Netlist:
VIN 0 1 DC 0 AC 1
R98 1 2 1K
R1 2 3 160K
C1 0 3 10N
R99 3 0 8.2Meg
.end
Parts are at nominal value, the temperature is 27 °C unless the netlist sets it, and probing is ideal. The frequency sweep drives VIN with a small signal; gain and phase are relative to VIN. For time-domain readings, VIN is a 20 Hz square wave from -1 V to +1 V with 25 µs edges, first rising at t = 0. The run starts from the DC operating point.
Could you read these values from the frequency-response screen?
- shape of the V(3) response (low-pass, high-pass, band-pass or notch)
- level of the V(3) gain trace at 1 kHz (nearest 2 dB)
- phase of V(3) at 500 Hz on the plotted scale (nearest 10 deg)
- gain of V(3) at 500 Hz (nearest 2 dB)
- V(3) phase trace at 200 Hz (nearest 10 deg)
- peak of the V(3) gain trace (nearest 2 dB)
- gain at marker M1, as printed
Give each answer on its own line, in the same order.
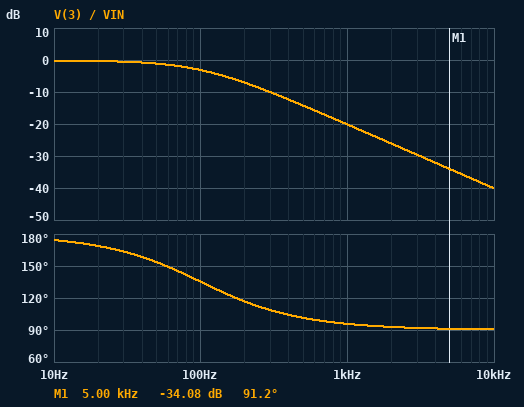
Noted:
low-pass
-20 dB
100 deg
-14 dB
120 deg
0 dB
-34.08 dB
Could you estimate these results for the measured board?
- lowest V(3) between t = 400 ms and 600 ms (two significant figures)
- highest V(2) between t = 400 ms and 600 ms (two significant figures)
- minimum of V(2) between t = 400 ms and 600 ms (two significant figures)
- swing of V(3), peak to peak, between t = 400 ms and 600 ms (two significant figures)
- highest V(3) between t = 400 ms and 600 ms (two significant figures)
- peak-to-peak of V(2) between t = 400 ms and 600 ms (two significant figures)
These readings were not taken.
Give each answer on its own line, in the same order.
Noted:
-980 mV
1.0 V
-1.0 V
2.0 V
980 mV
2.0 V
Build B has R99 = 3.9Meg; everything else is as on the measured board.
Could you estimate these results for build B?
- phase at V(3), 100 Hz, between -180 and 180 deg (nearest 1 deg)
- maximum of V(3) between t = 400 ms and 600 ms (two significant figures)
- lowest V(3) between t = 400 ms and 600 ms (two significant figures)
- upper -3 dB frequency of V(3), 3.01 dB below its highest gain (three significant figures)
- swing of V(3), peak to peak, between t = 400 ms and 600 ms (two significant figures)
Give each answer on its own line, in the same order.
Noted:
136 deg
960 mV
-960 mV
103 Hz
1.9 V
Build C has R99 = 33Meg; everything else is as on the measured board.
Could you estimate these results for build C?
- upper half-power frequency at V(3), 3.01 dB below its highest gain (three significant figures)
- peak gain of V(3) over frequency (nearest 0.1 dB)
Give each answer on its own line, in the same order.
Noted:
99.3 Hz
0 dB
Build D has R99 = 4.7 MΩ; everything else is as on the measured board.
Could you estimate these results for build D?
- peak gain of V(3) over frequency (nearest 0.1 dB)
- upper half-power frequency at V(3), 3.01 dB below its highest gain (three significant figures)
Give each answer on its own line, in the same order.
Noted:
-0.3 dB
102 Hz
